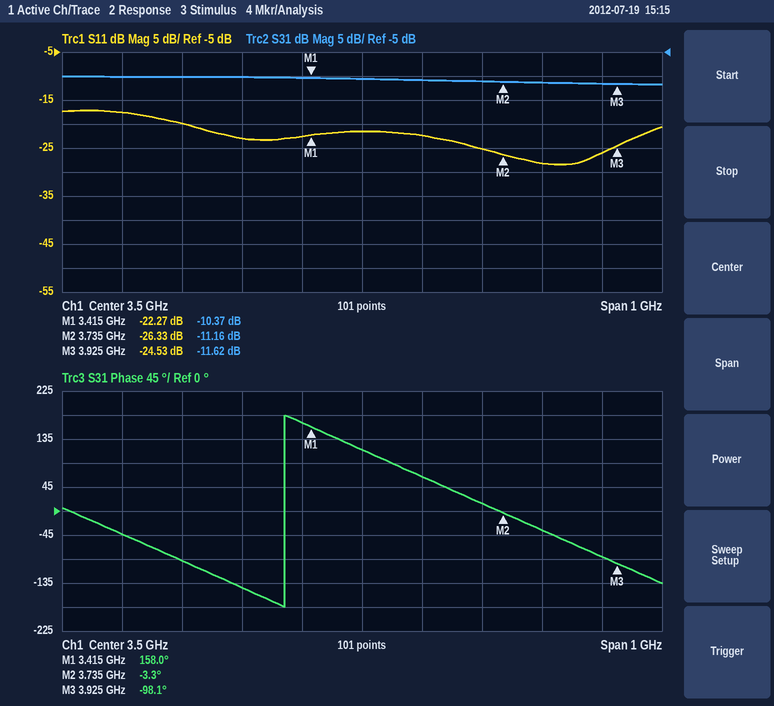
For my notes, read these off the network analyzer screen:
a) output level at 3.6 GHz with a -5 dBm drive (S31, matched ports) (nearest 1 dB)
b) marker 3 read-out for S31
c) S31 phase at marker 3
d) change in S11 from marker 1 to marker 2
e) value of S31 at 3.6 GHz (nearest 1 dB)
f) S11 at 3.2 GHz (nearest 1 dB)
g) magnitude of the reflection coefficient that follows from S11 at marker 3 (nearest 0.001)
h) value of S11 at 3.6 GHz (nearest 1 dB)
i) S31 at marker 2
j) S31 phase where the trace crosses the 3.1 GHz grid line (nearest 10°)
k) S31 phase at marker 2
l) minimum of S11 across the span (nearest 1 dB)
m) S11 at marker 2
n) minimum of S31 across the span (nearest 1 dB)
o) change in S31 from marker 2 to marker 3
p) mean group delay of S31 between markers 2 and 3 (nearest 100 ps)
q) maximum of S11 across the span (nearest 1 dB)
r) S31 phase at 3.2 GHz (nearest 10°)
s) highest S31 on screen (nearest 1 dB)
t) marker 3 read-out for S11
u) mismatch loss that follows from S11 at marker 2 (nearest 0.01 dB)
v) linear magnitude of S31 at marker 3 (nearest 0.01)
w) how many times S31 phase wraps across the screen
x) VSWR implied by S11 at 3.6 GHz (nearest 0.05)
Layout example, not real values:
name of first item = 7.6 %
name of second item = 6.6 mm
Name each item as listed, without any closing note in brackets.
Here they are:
output level at 3.6 GHz with a -5 dBm drive (S31, matched ports) = -16 dBm
marker 3 read-out for S31 = -11.62 dB
S31 phase at marker 3 = -98.1°
change in S11 from marker 1 to marker 2 = -4.06 dB
value of S31 at 3.6 GHz = -11 dB
S11 at 3.2 GHz = -20 dB
magnitude of the reflection coefficient that follows from S11 at marker 3 = 0.059
value of S11 at 3.6 GHz = -22 dB
S31 at marker 2 = -11.16 dB
S31 phase where the trace crosses the 3.1 GHz grid line = -40°
S31 phase at marker 2 = -3.3°
minimum of S11 across the span = -28 dB
S11 at marker 2 = -26.33 dB
minimum of S31 across the span = -12 dB
change in S31 from marker 2 to marker 3 = -0.46 dB
mean group delay of S31 between markers 2 and 3 = 1.4 ns
maximum of S11 across the span = -17 dB
S31 phase at 3.2 GHz = -90°
highest S31 on screen = -10 dB
marker 3 read-out for S11 = -24.53 dB
mismatch loss that follows from S11 at marker 2 = 0.01 dB
linear magnitude of S31 at marker 3 = 0.26
how many times S31 phase wraps across the screen = 1
VSWR implied by S11 at 3.6 GHz = 1.15
